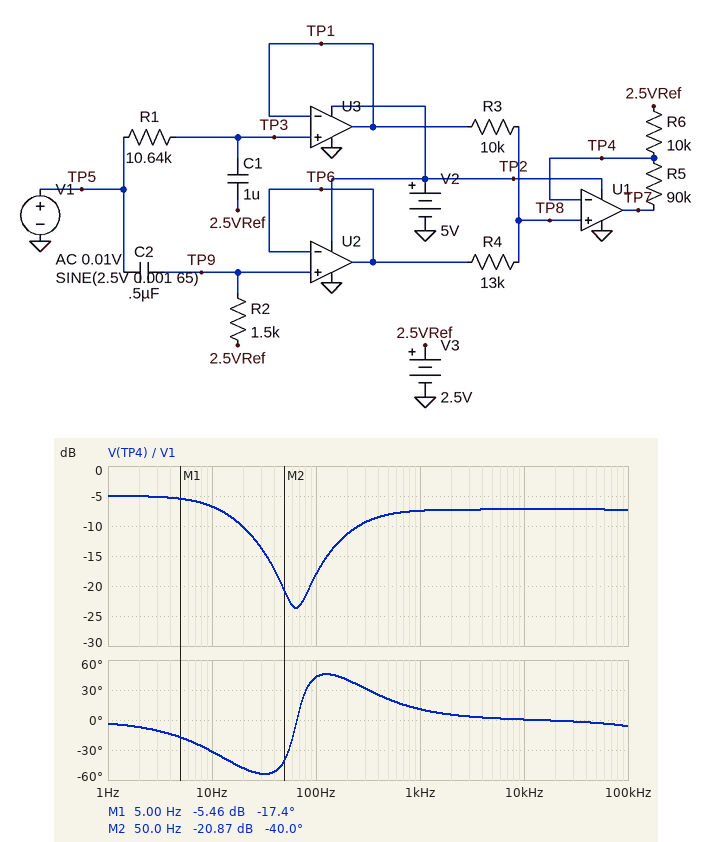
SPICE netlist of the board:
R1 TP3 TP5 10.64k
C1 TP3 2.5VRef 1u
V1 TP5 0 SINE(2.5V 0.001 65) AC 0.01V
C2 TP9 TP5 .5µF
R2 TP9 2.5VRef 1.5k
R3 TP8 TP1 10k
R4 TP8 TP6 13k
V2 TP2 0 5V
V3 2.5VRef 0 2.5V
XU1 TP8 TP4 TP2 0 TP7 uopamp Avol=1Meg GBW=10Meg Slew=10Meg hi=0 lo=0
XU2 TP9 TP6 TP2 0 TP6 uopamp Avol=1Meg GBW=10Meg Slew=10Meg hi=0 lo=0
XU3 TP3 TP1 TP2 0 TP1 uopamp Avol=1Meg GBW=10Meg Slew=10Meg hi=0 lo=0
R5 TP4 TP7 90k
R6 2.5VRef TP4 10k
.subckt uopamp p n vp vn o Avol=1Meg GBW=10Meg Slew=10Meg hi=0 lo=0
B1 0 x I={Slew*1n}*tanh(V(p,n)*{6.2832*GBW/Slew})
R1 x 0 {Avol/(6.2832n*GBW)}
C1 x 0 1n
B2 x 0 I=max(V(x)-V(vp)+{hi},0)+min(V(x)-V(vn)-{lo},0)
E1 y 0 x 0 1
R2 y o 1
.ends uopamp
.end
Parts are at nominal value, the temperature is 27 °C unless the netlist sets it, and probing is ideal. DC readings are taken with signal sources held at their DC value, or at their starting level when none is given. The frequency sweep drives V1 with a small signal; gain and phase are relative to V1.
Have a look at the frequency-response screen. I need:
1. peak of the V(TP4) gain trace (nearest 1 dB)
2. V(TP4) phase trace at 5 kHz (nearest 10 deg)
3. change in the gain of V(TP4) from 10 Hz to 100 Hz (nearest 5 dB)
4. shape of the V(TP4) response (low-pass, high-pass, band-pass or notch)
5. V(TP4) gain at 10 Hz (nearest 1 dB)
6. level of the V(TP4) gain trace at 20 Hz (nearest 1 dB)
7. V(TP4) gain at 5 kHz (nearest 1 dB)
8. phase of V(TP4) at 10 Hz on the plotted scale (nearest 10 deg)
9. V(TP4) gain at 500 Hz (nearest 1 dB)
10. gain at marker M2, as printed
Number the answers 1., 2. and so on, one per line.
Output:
1. -5 dB
2. 0 deg
3. -10 dB
4. notch
5. -7 dB
6. -10 dB
7. -7 dB
8. -30 deg
9. -8 dB
10. -20.87 dB
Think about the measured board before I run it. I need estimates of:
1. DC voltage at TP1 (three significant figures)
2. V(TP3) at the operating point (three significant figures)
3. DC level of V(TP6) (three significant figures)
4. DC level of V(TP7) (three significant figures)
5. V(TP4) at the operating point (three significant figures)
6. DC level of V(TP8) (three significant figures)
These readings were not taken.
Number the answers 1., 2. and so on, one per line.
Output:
1. 2.50 V
2. 2.50 V
3. 2.50 V
4. 2.50 V
5. 2.50 V
6. 2.50 V
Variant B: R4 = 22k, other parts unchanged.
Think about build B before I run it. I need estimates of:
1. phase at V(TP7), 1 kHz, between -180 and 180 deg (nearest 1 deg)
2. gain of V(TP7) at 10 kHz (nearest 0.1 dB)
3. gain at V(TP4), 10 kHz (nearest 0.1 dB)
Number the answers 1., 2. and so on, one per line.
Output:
1. 10 deg
2. 9.9 dB
3. -10.1 dB
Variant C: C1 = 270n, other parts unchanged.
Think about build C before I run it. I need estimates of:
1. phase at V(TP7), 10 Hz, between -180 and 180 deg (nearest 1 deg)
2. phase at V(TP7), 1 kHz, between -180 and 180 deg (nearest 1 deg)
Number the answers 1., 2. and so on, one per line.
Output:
1. -8 deg
2. 8 deg
